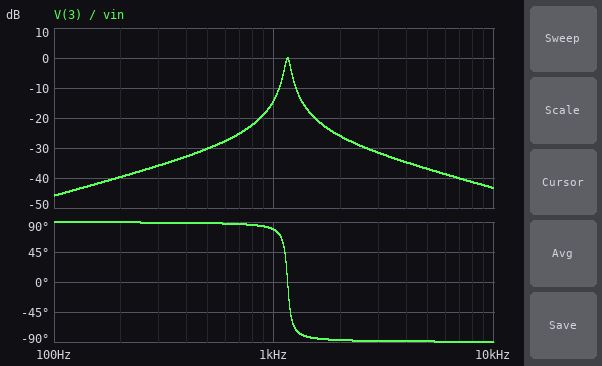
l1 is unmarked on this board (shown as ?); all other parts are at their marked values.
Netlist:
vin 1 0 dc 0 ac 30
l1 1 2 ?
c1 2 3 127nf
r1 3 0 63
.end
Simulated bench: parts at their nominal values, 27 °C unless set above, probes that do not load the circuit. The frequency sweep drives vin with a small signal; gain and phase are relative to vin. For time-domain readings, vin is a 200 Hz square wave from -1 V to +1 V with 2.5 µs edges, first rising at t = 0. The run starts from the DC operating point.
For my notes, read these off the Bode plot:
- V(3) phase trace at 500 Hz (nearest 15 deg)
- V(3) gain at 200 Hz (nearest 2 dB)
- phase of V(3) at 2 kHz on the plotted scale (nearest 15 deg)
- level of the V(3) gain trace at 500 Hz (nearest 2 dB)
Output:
90 deg
-40 dB
-90 deg
-30 dB
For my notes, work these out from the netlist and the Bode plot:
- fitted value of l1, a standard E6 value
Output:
150 mH
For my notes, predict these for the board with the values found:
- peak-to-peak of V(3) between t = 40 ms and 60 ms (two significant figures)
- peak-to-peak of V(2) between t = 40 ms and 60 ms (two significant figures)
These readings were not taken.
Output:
150 mV
4.5 V
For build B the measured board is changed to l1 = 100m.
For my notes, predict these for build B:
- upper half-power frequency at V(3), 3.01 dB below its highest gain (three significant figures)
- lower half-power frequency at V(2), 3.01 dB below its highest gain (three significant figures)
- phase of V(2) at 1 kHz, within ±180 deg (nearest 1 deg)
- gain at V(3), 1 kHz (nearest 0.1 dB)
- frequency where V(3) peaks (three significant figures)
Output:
1.46 kHz
1.36 kHz
-3 deg
-20.0 dB
1.41 kHz
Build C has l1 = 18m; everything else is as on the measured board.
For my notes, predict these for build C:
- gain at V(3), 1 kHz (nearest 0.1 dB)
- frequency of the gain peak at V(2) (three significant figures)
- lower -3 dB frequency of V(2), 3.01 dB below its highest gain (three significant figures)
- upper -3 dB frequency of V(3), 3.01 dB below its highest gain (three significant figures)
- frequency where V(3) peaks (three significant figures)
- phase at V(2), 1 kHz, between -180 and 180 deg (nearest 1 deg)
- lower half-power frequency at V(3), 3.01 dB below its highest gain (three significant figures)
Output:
-25.2 dB
3.31 kHz
3.01 kHz
3.62 kHz
3.33 kHz
0 deg
3.06 kHz
